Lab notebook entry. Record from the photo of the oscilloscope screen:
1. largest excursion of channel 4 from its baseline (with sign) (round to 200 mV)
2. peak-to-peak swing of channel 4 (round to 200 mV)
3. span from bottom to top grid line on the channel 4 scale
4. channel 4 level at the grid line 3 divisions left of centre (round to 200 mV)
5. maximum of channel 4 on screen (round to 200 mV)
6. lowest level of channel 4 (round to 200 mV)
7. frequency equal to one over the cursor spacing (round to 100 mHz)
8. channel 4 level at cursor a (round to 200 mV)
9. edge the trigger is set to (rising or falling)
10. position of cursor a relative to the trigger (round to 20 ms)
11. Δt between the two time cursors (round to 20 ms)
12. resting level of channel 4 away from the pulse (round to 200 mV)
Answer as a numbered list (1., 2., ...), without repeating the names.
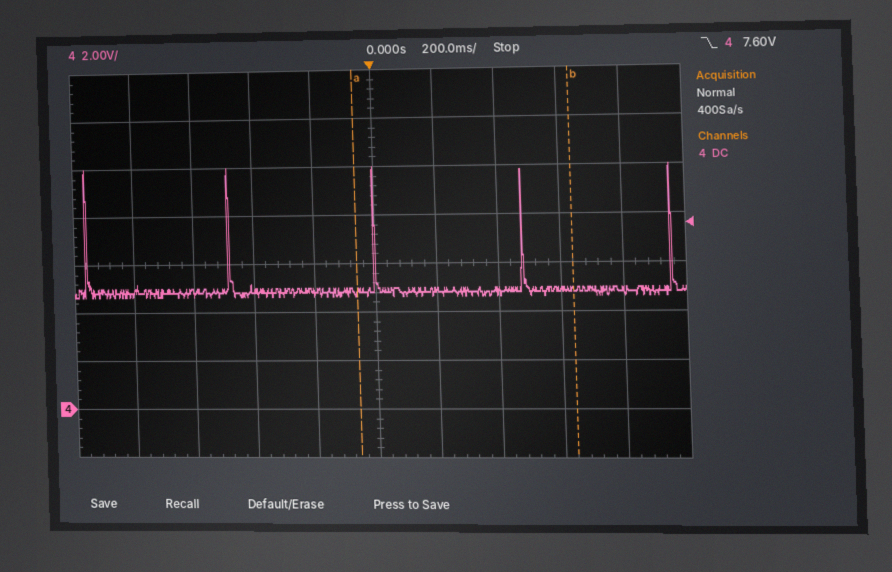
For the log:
1. +5.2 V
2. 5.4 V
3. 16 V
4. 4.8 V
5. 10.0 V
6. 4.6 V
7. 1.4 Hz
8. 4.8 V
9. falling
10. -60 ms
11. 700 ms
12. 4.8 V
